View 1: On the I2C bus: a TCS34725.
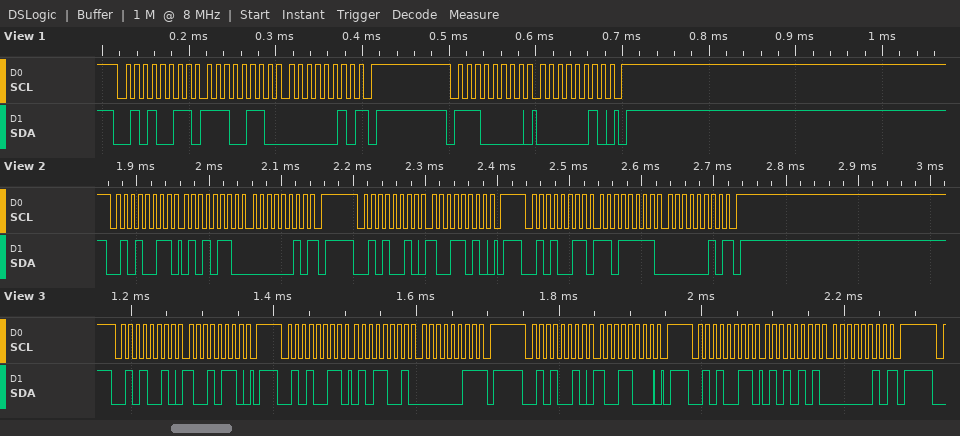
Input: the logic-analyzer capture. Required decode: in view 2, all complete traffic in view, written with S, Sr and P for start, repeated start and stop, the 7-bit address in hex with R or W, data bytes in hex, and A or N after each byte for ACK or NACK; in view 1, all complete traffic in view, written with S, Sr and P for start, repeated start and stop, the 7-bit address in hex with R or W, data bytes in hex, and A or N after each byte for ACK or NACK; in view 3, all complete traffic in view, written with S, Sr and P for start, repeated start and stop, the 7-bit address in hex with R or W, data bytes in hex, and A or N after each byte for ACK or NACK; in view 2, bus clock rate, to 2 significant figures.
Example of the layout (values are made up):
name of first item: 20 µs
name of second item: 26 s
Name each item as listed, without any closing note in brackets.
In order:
in view 2, all complete traffic in view, written with S, Sr and P for start, repeated start and stop, the 7-bit address in hex with R or W, data bytes in hex, and A or N after each byte for ACK or NACK: S 29R A 56 A 02 N P S 29W A 9A A P S 29R A DF A 02 N P
in view 1, all complete traffic in view, written with S, Sr and P for start, repeated start and stop, the 7-bit address in hex with R or W, data bytes in hex, and A or N after each byte for ACK or NACK: S 29R A E6 A 02 N P S 70W A 02 A P
in view 3, all complete traffic in view, written with S, Sr and P for start, repeated start and stop, the 7-bit address in hex with R or W, data bytes in hex, and A or N after each byte for ACK or NACK: S 29W A 96 A P S 29R A 59 A 03 N P S 29W A 98 A P S 29R A 55 A 02 N P
in view 2, bus clock rate, to 2 significant figures: 100 kHz
